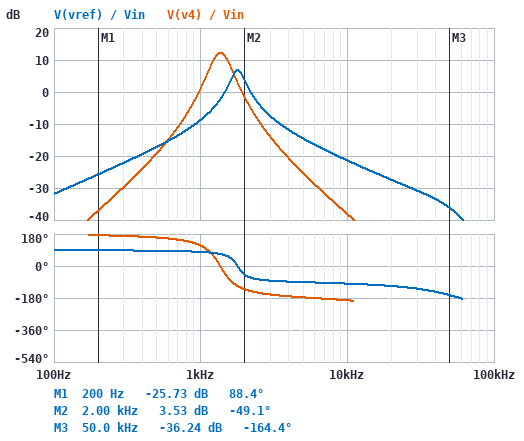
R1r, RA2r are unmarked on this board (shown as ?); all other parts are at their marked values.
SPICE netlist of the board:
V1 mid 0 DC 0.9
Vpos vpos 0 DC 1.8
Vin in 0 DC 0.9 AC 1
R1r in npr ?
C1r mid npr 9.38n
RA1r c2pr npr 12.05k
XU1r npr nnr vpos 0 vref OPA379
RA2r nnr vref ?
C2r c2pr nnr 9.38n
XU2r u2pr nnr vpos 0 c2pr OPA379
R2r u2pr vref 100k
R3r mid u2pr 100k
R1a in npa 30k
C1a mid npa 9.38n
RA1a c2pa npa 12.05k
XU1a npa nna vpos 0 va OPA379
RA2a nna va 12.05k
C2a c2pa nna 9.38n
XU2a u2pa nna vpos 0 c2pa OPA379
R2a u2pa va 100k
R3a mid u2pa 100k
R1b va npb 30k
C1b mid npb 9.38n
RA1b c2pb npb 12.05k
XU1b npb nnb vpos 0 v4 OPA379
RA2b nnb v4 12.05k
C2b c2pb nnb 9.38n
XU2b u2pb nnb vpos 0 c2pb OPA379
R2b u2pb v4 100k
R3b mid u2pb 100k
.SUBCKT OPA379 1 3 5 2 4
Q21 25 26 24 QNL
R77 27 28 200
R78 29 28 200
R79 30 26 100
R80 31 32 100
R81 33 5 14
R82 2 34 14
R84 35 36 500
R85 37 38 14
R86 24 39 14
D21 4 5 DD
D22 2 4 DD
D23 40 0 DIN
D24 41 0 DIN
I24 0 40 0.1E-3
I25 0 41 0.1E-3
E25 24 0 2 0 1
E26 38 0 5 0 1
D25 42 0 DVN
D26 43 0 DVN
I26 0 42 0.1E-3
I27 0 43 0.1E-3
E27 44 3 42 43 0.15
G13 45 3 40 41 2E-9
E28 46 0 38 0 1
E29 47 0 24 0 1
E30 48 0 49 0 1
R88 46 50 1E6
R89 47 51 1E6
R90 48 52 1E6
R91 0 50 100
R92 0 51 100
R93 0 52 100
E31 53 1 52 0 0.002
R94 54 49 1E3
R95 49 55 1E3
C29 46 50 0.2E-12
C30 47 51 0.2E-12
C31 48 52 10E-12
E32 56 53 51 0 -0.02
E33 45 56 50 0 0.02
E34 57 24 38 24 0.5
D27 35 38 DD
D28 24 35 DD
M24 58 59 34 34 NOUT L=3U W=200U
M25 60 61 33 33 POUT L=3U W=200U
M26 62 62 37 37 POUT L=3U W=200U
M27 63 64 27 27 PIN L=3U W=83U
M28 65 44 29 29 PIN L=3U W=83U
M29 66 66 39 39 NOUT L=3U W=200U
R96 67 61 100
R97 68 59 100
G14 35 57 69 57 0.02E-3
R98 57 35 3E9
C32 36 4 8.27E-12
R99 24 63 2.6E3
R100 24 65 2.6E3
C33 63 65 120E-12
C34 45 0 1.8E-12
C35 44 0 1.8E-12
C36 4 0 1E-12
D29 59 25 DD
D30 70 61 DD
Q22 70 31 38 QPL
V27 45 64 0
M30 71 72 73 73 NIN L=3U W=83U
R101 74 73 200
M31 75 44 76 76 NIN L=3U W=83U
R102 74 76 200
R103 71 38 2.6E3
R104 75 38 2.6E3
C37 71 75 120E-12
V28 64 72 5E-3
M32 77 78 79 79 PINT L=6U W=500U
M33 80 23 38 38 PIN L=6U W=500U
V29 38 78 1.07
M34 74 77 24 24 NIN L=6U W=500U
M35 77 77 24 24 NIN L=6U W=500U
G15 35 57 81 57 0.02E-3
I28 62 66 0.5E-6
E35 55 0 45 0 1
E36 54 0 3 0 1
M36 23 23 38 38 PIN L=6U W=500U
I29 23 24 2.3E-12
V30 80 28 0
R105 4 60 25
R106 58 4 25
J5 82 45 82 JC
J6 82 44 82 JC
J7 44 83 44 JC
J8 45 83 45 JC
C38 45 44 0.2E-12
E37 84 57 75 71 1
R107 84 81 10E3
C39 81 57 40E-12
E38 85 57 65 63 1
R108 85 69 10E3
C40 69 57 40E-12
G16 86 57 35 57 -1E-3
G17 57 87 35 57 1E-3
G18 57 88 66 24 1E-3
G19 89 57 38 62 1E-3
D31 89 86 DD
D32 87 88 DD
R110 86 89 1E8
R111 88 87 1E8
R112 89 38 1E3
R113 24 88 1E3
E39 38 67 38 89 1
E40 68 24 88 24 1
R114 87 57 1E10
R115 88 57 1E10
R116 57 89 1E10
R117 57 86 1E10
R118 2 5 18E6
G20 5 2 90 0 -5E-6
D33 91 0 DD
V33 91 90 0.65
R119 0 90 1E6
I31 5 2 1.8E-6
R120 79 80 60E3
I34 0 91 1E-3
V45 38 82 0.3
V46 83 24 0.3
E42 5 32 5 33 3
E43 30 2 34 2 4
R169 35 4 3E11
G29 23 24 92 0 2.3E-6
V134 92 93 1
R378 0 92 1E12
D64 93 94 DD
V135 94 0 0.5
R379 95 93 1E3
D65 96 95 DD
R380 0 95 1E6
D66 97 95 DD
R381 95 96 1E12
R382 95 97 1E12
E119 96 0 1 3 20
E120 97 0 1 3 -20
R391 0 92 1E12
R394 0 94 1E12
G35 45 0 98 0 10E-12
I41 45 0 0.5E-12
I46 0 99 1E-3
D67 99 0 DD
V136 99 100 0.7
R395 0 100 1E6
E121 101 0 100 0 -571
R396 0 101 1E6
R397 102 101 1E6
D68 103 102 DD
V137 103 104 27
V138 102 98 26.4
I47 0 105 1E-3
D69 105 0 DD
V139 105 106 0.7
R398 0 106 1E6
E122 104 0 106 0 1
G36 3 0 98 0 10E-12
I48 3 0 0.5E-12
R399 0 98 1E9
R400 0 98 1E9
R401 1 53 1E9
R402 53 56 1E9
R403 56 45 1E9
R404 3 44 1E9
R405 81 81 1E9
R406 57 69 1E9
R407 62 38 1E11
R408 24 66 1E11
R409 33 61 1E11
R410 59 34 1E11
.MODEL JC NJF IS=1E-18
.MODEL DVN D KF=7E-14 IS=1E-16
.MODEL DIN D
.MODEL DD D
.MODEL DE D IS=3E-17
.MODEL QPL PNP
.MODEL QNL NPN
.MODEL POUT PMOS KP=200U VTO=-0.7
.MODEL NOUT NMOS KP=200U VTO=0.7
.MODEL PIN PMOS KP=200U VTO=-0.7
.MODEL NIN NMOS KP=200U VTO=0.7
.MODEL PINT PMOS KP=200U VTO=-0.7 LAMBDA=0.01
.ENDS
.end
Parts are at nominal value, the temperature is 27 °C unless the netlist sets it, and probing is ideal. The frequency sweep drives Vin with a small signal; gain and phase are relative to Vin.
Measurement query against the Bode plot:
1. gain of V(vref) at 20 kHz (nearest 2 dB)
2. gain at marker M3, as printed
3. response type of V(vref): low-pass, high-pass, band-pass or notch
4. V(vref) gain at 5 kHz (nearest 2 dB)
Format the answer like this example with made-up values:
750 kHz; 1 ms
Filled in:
-28 dB; -36.24 dB; band-pass; -14 dB
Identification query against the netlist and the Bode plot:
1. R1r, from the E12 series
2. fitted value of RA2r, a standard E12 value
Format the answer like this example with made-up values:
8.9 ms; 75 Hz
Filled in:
39 kΩ; 6.8 kΩ
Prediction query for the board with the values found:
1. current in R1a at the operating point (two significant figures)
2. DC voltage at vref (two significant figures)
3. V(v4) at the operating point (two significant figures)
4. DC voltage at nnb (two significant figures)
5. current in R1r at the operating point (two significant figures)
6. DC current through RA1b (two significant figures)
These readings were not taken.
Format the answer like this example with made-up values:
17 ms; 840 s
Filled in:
170 nA; 890 mV; 890 mV; 890 mV; 130 nA; 170 nA
